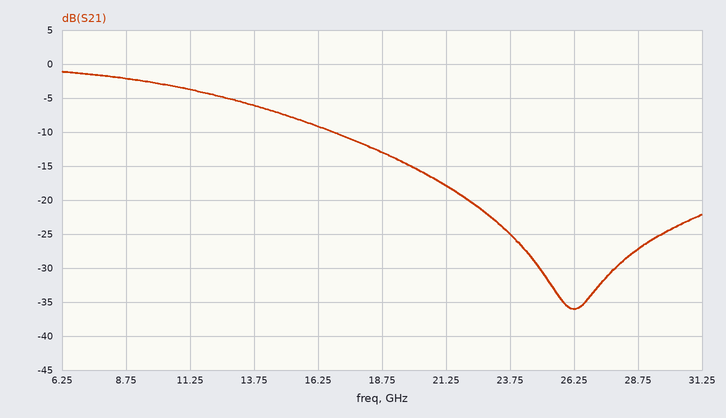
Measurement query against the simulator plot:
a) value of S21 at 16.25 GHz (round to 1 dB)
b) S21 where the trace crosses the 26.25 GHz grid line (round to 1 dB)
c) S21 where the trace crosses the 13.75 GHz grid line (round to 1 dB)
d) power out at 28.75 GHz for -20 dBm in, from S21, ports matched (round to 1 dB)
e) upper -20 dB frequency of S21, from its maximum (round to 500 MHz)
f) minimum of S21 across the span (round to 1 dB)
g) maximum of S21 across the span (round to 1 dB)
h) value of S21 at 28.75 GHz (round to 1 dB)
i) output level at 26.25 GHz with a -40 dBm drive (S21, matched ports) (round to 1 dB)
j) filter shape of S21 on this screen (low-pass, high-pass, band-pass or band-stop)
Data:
-9 dB
-36 dB
-6 dB
-47 dBm
22.5 GHz
-36 dB
-1 dB
-27 dB
-76 dBm
low-pass
